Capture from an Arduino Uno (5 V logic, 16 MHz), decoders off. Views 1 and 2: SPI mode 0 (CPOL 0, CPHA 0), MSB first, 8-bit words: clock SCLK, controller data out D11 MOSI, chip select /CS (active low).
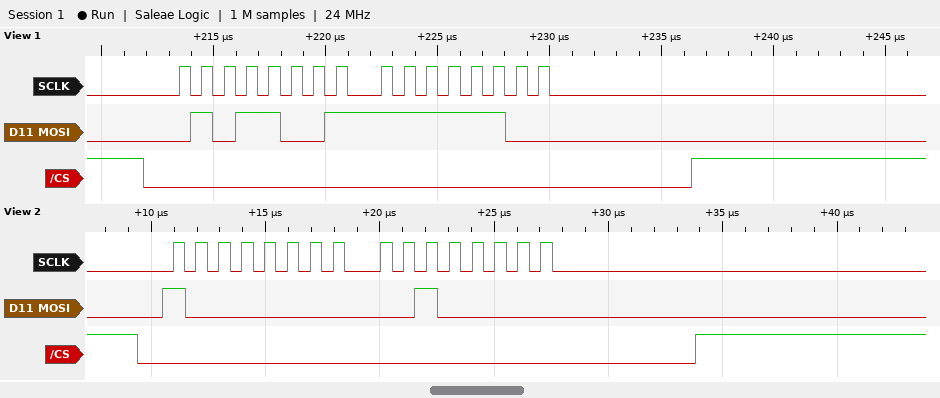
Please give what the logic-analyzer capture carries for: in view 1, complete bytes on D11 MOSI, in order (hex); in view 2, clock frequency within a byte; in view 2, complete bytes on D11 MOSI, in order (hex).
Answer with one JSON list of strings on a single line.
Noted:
["59 FC", "1 MHz", "80 20"]
